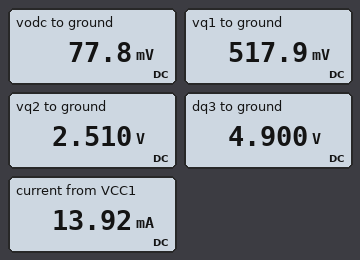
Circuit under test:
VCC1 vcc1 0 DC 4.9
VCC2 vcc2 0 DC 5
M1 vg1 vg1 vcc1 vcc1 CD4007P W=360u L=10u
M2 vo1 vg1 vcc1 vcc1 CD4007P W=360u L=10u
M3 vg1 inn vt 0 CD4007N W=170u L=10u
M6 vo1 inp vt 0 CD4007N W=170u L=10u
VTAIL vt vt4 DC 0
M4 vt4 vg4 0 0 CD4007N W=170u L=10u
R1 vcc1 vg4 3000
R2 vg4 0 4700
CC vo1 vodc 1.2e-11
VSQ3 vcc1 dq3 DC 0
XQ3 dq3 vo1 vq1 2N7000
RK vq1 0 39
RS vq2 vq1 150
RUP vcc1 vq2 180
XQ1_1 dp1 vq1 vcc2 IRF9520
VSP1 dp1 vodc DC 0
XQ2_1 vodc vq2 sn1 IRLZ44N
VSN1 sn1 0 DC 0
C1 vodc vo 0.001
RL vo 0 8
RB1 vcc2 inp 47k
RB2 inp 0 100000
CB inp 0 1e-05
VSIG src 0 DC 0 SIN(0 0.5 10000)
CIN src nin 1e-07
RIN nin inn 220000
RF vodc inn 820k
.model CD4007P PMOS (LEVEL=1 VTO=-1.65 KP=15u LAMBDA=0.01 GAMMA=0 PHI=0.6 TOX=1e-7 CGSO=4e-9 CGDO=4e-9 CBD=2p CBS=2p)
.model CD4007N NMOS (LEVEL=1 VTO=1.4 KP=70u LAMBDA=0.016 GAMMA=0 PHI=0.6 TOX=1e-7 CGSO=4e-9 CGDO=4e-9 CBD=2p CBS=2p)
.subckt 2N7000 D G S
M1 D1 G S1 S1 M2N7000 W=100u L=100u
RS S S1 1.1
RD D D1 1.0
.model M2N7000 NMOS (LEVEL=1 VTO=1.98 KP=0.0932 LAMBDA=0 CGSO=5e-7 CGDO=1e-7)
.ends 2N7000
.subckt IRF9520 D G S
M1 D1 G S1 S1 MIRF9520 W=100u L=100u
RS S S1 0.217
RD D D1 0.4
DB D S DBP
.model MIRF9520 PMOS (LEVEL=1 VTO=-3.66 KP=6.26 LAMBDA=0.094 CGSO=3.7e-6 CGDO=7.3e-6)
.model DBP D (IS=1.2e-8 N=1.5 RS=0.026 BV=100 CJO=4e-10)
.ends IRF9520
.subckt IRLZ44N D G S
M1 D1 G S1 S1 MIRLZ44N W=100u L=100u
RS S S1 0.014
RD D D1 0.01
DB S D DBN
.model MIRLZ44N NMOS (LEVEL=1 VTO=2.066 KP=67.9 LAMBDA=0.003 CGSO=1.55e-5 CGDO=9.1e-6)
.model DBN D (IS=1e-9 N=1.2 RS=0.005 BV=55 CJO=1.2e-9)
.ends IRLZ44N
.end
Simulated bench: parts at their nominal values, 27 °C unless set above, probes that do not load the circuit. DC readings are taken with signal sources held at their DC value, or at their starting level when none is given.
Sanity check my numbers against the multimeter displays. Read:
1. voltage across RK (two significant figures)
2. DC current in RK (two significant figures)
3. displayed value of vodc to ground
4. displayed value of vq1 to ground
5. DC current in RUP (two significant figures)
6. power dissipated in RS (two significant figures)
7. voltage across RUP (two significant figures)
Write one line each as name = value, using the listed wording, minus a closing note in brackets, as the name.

voltage across RK = 520 mV
DC current in RK = 13 mA
displayed value of vodc to ground = 77.8 mV
displayed value of vq1 to ground = 517.9 mV
DC current in RUP = 13 mA
power dissipated in RS = 26 mW
voltage across RUP = 2.4 V
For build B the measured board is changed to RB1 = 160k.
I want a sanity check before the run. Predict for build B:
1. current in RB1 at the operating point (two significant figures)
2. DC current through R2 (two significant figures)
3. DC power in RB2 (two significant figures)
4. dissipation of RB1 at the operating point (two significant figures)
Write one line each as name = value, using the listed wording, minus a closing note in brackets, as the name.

current in RB1 at the operating point = 19 µA
DC current through R2 = 640 µA
DC power in RB2 = 37 µW
dissipation of RB1 at the operating point = 59 µW
